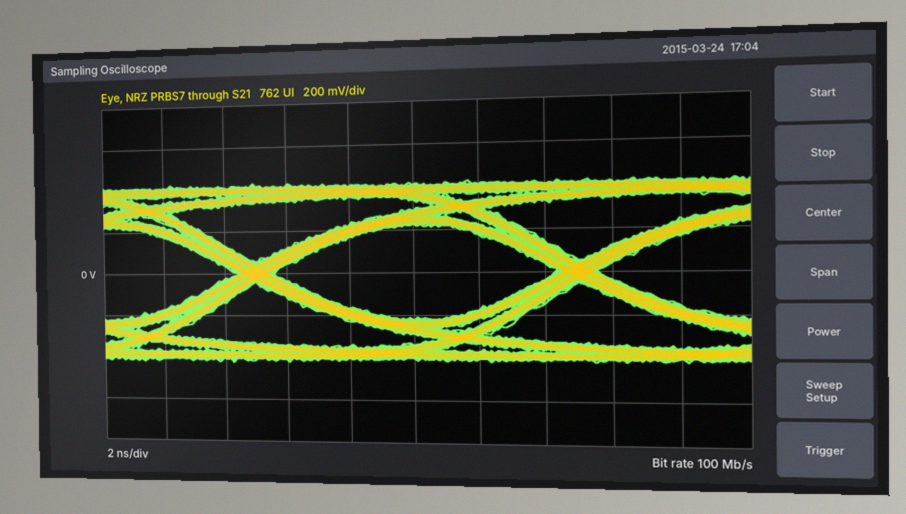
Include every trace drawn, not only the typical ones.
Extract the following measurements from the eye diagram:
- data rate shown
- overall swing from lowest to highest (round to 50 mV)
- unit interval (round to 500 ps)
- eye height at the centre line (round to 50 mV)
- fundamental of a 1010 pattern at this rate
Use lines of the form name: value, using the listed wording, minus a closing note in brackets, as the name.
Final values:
data rate shown: 100 Mb/s
overall swing from lowest to highest: 850 mV
unit interval: 10.0 ns
eye height at the centre line: 450 mV
fundamental of a 1010 pattern at this rate: 50 MHz
